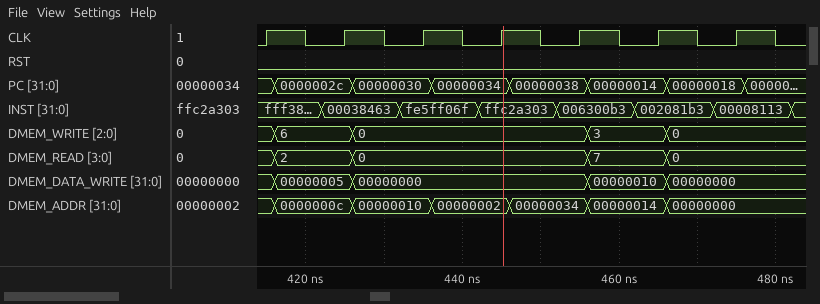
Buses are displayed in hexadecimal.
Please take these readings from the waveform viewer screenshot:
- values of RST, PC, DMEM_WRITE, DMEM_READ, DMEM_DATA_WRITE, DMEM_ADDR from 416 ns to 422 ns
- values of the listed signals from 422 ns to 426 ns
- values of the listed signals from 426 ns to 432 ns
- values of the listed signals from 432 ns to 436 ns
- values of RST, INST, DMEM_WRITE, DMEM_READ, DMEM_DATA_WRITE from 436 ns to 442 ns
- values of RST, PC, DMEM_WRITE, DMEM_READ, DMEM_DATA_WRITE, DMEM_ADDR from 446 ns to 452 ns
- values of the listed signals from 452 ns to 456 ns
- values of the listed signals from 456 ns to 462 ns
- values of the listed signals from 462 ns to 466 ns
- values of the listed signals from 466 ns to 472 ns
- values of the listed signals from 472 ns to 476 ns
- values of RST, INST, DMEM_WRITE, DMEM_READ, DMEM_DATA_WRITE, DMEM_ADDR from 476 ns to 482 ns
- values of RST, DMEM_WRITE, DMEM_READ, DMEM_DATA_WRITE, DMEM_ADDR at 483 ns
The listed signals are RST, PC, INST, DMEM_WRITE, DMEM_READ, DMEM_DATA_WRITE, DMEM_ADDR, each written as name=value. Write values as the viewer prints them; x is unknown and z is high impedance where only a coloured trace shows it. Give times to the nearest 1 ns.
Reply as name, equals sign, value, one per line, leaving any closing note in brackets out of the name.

values of RST, PC, DMEM_WRITE, DMEM_READ, DMEM_DATA_WRITE, DMEM_ADDR from 416 ns to 422 ns = RST=0, PC=0000002c, DMEM_WRITE=6, DMEM_READ=2, DMEM_DATA_WRITE=00000005, DMEM_ADDR=0000000c
values of the listed signals from 422 ns to 426 ns = RST=0, PC=0000002c, INST=00038463, DMEM_WRITE=6, DMEM_READ=2, DMEM_DATA_WRITE=00000005, DMEM_ADDR=0000000c
values of the listed signals from 426 ns to 432 ns = RST=0, PC=00000030, INST=00038463, DMEM_WRITE=0, DMEM_READ=0, DMEM_DATA_WRITE=00000000, DMEM_ADDR=00000010
values of the listed signals from 432 ns to 436 ns = RST=0, PC=00000030, INST=fe5ff06f, DMEM_WRITE=0, DMEM_READ=0, DMEM_DATA_WRITE=00000000, DMEM_ADDR=00000010
values of RST, INST, DMEM_WRITE, DMEM_READ, DMEM_DATA_WRITE from 436 ns to 442 ns = RST=0, INST=fe5ff06f, DMEM_WRITE=0, DMEM_READ=0, DMEM_DATA_WRITE=00000000
values of RST, PC, DMEM_WRITE, DMEM_READ, DMEM_DATA_WRITE, DMEM_ADDR from 446 ns to 452 ns = RST=0, PC=00000038, DMEM_WRITE=0, DMEM_READ=0, DMEM_DATA_WRITE=00000000, DMEM_ADDR=00000034
values of the listed signals from 452 ns to 456 ns = RST=0, PC=00000038, INST=006300b3, DMEM_WRITE=0, DMEM_READ=0, DMEM_DATA_WRITE=00000000, DMEM_ADDR=00000034
values of the listed signals from 456 ns to 462 ns = RST=0, PC=00000014, INST=006300b3, DMEM_WRITE=3, DMEM_READ=7, DMEM_DATA_WRITE=00000010, DMEM_ADDR=00000014
values of the listed signals from 462 ns to 466 ns = RST=0, PC=00000014, INST=002081b3, DMEM_WRITE=3, DMEM_READ=7, DMEM_DATA_WRITE=00000010, DMEM_ADDR=00000014
values of the listed signals from 466 ns to 472 ns = RST=0, PC=00000018, INST=002081b3, DMEM_WRITE=0, DMEM_READ=0, DMEM_DATA_WRITE=00000000, DMEM_ADDR=00000000
values of the listed signals from 472 ns to 476 ns = RST=0, PC=00000018, INST=00008113, DMEM_WRITE=0, DMEM_READ=0, DMEM_DATA_WRITE=00000000, DMEM_ADDR=00000000
values of RST, INST, DMEM_WRITE, DMEM_READ, DMEM_DATA_WRITE, DMEM_ADDR from 476 ns to 482 ns = RST=0, INST=00008113, DMEM_WRITE=0, DMEM_READ=0, DMEM_DATA_WRITE=00000000, DMEM_ADDR=00000000
values of RST, DMEM_WRITE, DMEM_READ, DMEM_DATA_WRITE, DMEM_ADDR at 483 ns = RST=0, DMEM_WRITE=0, DMEM_READ=0, DMEM_DATA_WRITE=00000000, DMEM_ADDR=00000000
